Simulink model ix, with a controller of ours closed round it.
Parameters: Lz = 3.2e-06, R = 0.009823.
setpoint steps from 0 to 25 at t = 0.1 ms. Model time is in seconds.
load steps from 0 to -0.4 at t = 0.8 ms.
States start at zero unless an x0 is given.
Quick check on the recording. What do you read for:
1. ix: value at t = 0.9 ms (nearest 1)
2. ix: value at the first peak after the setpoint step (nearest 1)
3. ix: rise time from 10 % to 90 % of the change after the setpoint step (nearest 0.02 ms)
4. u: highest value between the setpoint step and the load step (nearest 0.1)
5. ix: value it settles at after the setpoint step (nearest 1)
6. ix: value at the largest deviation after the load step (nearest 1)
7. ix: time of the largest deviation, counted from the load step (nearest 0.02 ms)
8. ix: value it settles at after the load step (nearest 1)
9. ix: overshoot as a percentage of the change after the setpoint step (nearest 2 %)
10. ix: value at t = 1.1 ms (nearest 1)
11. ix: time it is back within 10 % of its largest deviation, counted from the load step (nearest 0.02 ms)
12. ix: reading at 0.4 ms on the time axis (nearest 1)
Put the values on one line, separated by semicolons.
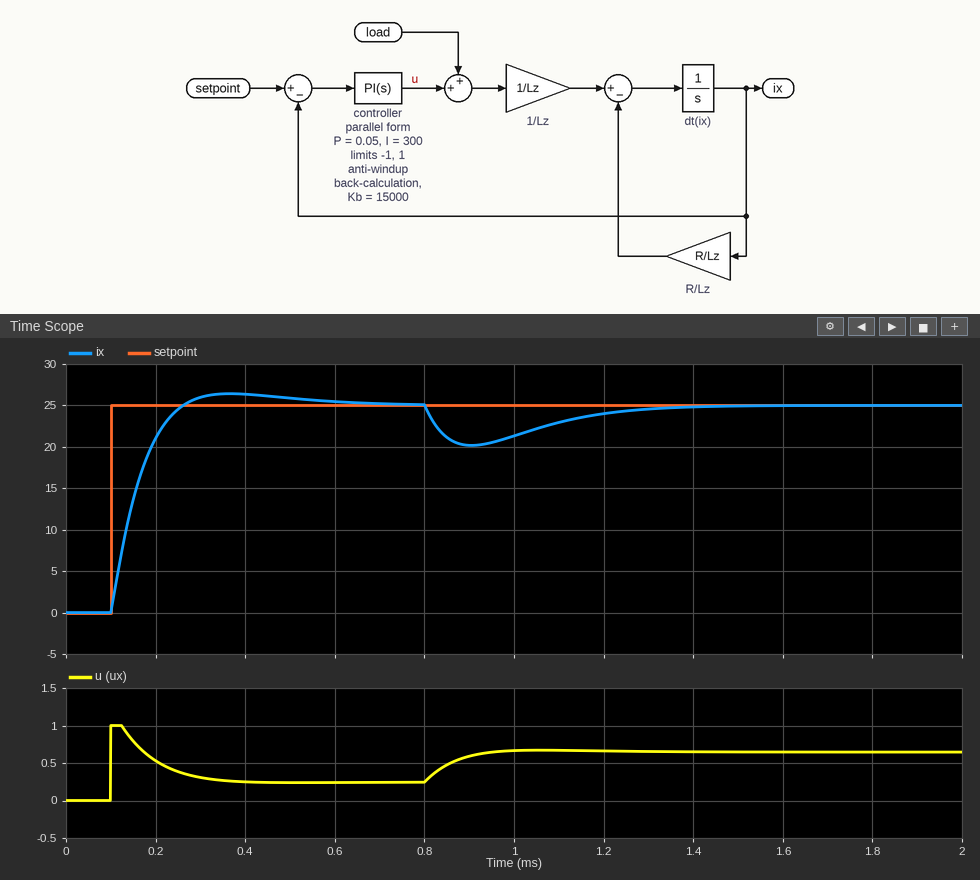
20; 26; 0.10 ms; 1.0; 25; 20; 0.10 ms; 25; 6 %; 23; 0.48 ms; 26
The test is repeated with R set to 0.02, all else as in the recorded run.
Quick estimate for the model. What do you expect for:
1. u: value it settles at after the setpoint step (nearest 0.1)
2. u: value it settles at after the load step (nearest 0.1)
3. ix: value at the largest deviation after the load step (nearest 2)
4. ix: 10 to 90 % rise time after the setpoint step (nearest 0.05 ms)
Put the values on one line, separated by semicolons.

0.5; 0.9; 20; 0.15 ms
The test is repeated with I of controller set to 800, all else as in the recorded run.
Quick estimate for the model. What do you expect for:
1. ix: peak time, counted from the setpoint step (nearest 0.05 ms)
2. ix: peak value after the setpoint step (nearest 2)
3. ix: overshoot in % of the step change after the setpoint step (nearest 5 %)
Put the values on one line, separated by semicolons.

0.15 ms; 30; 20 %
